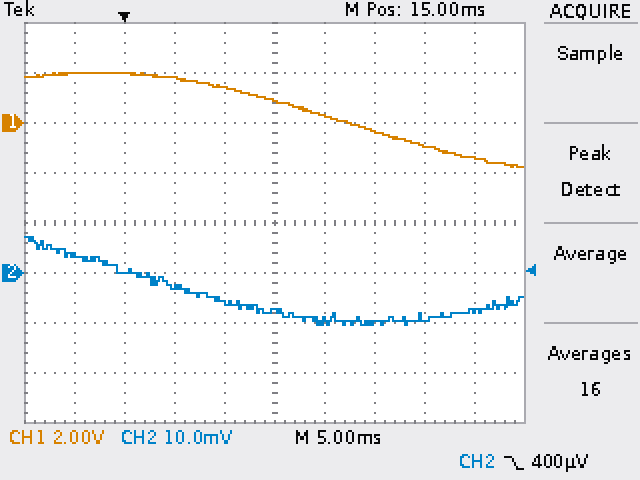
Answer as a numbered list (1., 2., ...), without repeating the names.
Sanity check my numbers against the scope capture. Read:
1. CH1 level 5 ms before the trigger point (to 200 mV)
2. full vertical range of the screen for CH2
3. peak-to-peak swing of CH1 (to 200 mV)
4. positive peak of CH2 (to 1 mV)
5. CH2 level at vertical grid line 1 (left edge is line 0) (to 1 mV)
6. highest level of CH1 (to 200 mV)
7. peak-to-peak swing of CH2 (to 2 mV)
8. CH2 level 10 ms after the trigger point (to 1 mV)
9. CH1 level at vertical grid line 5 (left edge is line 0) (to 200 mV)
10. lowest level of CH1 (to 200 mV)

1. 2.0 V
2. 80 mV
3. 3.8 V
4. 7 mV
5. 4 mV
6. 2.0 V
7. 18 mV
8. -6 mV
9. 800 mV
10. -1.8 V
